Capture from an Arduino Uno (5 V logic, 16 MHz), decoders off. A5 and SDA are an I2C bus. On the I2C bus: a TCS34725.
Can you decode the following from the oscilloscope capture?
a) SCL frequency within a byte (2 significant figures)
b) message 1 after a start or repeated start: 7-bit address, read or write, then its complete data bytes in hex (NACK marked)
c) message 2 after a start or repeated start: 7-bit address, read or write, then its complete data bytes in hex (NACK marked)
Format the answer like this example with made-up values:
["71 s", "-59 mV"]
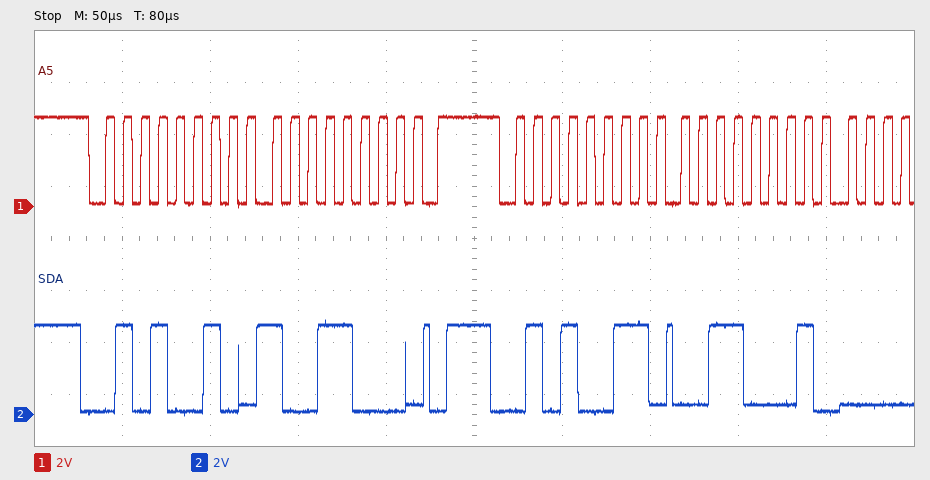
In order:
["100 kHz", "0x29 write: 98", "0x29 read: 31"]
